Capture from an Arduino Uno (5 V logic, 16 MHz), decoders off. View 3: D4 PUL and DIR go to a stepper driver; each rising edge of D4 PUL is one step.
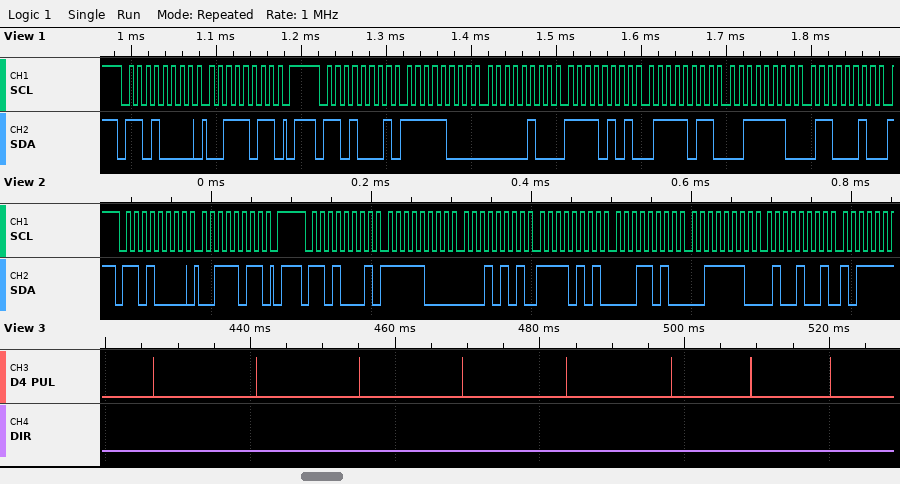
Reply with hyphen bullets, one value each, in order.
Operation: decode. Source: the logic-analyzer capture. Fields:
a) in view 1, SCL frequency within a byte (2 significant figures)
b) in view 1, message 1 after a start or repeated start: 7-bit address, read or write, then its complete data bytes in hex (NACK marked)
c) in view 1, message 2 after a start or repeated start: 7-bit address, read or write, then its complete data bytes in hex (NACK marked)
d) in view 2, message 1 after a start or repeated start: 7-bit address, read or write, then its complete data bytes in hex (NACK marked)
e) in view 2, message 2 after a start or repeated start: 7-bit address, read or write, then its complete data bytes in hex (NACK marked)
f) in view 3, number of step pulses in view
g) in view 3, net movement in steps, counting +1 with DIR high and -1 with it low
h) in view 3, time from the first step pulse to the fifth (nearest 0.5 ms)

- 100 kHz
- 0x68 write: 3B
- 0x68 read: F8 04 F5 7B 3E 62
- 0x68 write: 3B
- 0x68 read: F8 15 F5 1A 3E 49
- 8
- -8
- 57.0 ms
